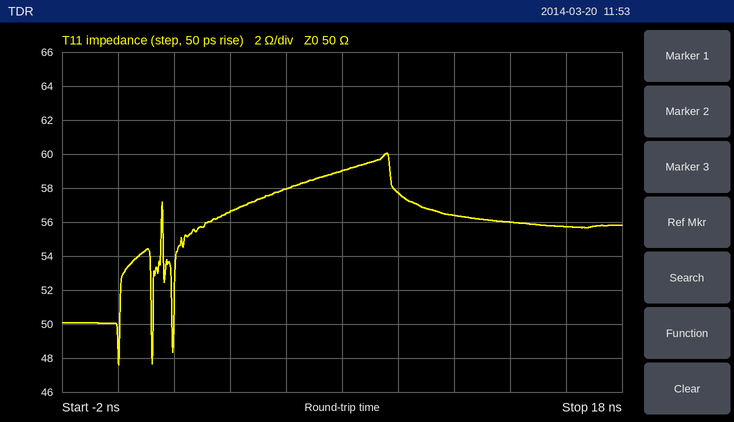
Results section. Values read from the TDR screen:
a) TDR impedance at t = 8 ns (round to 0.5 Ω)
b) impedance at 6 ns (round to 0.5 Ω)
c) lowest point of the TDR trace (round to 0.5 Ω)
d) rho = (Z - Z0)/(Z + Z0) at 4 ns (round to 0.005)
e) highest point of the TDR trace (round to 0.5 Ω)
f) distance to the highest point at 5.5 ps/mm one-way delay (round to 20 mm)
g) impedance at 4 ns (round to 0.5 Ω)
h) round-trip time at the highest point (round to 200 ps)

59.0 Ω
58.0 Ω
47.5 Ω
+0.060
60.0 Ω
880 mm
56.5 Ω
9.6 ns
